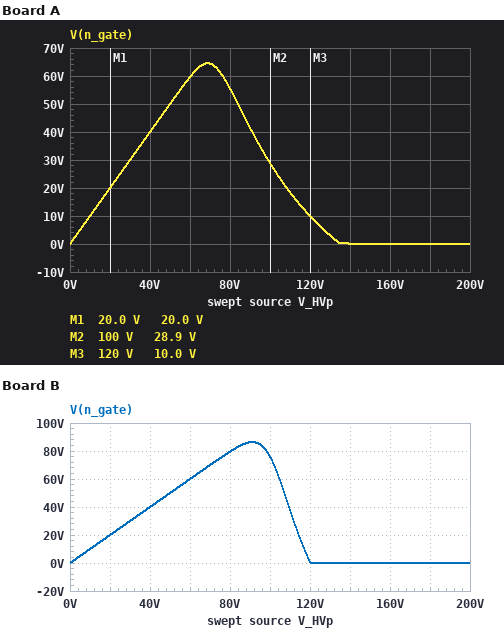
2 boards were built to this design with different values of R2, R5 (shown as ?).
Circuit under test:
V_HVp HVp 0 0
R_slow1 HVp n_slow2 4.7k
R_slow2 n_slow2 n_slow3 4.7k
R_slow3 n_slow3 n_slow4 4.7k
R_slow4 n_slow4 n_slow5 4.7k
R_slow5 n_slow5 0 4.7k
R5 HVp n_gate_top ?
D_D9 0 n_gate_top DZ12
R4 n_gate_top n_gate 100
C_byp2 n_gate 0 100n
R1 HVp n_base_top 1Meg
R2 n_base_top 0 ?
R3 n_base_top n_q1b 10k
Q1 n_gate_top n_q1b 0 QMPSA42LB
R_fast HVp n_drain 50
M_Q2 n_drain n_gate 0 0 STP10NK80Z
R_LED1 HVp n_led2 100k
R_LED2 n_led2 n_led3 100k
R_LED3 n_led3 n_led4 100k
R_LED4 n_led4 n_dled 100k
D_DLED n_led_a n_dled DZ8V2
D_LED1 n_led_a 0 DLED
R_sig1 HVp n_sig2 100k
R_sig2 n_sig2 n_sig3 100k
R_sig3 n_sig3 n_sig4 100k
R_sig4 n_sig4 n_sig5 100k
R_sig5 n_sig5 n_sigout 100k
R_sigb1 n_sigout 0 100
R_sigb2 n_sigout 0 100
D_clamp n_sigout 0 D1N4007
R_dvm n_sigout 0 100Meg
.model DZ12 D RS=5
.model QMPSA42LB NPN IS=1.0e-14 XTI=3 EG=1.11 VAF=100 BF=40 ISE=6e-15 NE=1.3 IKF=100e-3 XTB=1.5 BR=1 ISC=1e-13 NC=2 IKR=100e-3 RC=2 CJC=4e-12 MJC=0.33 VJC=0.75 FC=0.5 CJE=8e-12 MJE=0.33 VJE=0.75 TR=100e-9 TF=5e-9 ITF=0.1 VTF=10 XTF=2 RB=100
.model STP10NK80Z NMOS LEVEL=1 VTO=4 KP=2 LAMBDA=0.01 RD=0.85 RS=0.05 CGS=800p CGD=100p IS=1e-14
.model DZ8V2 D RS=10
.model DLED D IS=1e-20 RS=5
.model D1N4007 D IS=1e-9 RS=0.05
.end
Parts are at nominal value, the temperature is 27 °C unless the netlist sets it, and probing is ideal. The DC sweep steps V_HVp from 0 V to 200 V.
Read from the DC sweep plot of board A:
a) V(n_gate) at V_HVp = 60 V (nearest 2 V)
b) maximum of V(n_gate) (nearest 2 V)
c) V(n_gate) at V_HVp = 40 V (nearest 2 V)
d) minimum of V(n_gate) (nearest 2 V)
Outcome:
60 V
64 V
40 V
0 V
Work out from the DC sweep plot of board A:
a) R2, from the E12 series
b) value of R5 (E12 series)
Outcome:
8.2 kΩ
150 kΩ
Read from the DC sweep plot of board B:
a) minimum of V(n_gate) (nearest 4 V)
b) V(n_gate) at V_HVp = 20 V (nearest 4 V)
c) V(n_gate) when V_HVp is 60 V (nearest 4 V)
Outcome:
0 V
20 V
60 V
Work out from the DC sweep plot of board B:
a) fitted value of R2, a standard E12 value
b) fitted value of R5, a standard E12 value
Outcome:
5.6 kΩ
820 kΩ
